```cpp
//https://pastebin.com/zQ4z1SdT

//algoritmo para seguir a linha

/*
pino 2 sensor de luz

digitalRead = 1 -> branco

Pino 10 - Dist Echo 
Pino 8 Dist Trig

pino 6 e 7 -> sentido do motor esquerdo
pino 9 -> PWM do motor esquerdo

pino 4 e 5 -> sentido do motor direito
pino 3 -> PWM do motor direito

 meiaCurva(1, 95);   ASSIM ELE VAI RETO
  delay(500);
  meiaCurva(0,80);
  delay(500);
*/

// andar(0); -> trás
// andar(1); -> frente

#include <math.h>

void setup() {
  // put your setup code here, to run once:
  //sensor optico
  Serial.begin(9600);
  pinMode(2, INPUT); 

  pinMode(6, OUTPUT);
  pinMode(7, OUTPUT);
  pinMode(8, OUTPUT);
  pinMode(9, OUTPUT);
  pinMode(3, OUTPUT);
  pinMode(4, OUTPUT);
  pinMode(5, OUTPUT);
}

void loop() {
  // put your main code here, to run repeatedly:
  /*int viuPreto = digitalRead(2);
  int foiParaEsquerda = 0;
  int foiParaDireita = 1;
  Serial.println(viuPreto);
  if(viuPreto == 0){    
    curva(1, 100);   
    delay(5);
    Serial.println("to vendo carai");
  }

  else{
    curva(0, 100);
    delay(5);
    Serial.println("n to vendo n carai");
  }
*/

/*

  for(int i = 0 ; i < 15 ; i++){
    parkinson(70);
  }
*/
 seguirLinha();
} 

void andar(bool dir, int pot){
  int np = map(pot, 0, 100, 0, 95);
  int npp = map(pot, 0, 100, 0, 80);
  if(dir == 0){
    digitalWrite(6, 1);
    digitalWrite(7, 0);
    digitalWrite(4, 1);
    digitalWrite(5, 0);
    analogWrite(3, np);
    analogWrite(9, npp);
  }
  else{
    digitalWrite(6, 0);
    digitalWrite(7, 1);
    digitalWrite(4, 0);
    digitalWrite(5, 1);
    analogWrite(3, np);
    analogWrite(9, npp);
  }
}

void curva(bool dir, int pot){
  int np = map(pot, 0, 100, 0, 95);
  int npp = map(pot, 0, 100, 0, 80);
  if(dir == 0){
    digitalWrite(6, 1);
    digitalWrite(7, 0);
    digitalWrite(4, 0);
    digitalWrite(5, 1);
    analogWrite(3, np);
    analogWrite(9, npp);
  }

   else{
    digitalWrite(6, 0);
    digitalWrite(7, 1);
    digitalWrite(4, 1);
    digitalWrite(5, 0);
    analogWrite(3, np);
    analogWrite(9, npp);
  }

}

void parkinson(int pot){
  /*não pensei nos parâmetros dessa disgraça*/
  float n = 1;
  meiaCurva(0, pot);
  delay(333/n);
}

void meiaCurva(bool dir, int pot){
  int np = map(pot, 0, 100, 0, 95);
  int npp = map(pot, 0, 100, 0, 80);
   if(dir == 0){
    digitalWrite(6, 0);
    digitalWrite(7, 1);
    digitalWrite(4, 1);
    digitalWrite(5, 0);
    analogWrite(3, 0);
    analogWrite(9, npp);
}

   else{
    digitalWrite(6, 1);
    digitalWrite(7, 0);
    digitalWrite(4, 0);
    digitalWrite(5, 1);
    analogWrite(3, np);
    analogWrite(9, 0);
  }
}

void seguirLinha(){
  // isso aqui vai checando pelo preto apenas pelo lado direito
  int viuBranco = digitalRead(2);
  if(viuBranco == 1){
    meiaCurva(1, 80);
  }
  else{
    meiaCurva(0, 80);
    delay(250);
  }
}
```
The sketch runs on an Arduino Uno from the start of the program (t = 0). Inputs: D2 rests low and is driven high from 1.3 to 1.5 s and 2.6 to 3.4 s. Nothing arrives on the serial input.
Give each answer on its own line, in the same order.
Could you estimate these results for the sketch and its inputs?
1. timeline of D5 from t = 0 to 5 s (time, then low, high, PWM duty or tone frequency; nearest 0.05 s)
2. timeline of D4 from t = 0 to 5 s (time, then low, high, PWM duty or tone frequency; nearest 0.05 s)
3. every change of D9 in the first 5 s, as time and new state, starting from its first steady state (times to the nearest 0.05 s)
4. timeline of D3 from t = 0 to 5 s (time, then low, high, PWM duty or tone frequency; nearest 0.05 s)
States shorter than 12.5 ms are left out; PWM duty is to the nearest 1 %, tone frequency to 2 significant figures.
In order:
0 s low; 2.75 s high; 3.4 s low
0 s high; 2.75 s low; 3.4 s high
0 s PWM 25 %; 2.75 s low; 3.4 s PWM 25 %
0 s low; 2.75 s PWM 30 %; 3.4 s low
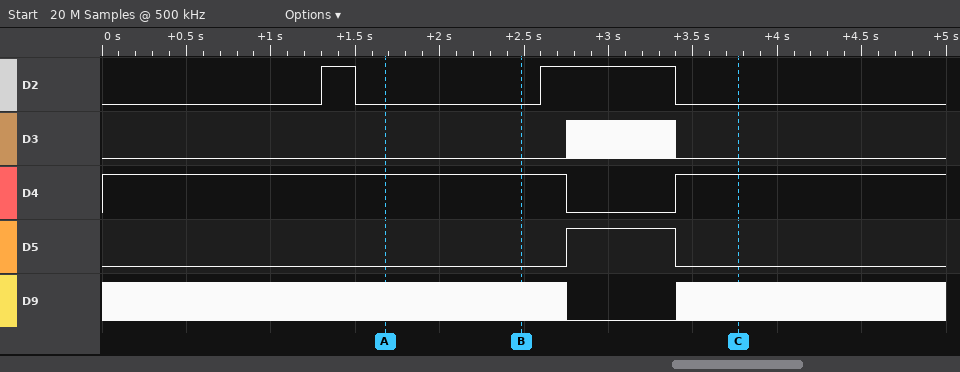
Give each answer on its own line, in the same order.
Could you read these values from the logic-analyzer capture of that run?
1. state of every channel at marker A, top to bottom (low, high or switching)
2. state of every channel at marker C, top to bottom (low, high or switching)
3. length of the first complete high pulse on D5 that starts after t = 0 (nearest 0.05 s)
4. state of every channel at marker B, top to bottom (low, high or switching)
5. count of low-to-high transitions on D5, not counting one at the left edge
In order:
D2 low, D3 low, D4 high, D5 low, D9 switching
D2 low, D3 low, D4 high, D5 low, D9 switching
0.65 s
D2 low, D3 low, D4 high, D5 low, D9 switching
1
